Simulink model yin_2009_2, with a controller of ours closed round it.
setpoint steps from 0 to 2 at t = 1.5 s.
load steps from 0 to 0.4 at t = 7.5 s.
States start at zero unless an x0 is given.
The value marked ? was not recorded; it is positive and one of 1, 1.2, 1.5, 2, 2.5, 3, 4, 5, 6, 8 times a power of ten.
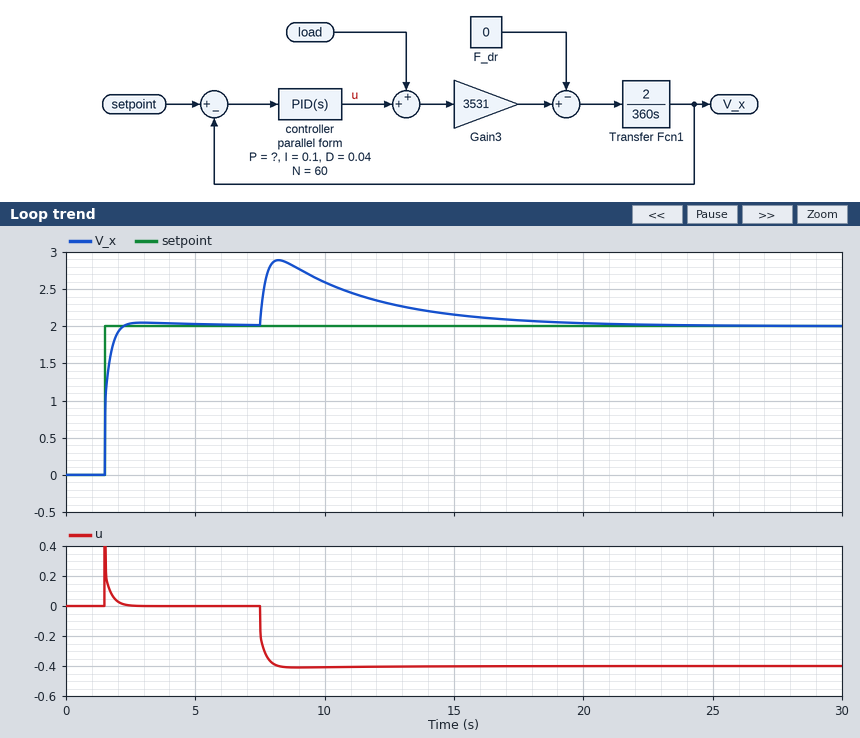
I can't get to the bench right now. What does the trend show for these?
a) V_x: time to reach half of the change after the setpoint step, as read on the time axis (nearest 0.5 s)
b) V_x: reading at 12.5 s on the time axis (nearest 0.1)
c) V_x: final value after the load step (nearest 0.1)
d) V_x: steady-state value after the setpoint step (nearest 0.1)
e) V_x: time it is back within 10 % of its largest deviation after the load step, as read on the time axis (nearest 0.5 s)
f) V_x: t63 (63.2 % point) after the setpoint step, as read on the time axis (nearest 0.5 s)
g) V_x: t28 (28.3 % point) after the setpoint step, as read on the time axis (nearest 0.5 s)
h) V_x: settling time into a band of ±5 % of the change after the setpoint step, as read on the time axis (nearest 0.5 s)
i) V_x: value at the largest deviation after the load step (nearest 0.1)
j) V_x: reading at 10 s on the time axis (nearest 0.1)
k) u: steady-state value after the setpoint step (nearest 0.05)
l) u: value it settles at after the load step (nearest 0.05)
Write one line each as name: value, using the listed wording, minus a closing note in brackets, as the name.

V_x: time to reach half of the change after the setpoint step, as read on the time axis: 1.5 s
V_x: reading at 12.5 s on the time axis: 2.3
V_x: final value after the load step: 2.0
V_x: steady-state value after the setpoint step: 2.0
V_x: time it is back within 10 % of its largest deviation after the load step, as read on the time axis: 17.0 s
V_x: t63 (63.2 % point) after the setpoint step, as read on the time axis: 1.5 s
V_x: t28 (28.3 % point) after the setpoint step, as read on the time axis: 1.5 s
V_x: settling time into a band of ±5 % of the change after the setpoint step, as read on the time axis: 2.0 s
V_x: value at the largest deviation after the load step: 2.9
V_x: reading at 10 s on the time axis: 2.6
u: steady-state value after the setpoint step: 0.00
u: value it settles at after the load step: -0.40
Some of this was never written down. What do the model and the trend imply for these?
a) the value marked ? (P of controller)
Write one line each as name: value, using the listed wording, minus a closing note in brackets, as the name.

the value marked ?: 0.4
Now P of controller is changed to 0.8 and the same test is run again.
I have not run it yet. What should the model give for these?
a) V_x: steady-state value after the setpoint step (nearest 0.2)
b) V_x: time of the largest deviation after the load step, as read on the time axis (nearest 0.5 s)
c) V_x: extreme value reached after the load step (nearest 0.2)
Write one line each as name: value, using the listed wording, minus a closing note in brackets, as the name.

V_x: steady-state value after the setpoint step: 2.0
V_x: time of the largest deviation after the load step, as read on the time axis: 8.0 s
V_x: extreme value reached after the load step: 2.4
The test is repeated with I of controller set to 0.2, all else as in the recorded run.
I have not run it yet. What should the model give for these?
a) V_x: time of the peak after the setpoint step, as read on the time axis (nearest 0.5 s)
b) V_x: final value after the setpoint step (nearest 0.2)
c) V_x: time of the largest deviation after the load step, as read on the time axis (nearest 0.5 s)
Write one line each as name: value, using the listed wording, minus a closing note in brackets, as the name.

V_x: time of the peak after the setpoint step, as read on the time axis: 2.5 s
V_x: final value after the setpoint step: 2.0
V_x: time of the largest deviation after the load step, as read on the time axis: 8.0 s
